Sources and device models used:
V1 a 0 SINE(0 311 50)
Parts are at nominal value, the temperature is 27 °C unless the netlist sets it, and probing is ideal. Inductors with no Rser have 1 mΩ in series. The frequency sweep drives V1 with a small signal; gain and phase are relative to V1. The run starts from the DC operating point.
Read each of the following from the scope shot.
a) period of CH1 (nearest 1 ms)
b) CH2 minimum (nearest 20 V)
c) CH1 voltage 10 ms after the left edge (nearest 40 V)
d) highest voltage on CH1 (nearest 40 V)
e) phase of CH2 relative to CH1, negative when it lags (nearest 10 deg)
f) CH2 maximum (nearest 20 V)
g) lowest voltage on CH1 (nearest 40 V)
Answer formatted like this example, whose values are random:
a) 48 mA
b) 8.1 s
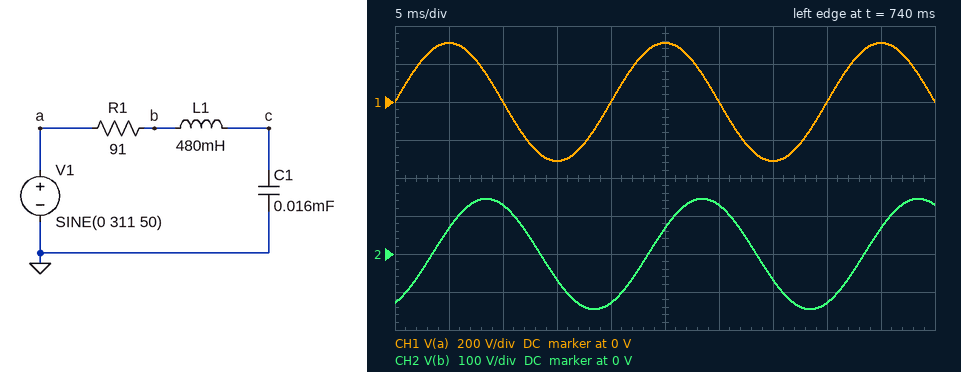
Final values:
a) 20 ms
b) -140 V
c) 0 V
d) 320 V
e) -60 deg
f) 140 V
g) -320 V
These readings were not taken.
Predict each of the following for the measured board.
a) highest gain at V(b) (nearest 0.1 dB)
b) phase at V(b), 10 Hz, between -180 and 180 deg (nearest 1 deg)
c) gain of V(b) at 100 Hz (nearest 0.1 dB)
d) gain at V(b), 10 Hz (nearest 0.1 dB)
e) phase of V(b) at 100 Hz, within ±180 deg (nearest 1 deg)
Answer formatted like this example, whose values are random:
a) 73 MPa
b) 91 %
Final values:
a) 0 dB
b) -5 deg
c) -0.8 dB
d) 0 dB
e) 24 deg
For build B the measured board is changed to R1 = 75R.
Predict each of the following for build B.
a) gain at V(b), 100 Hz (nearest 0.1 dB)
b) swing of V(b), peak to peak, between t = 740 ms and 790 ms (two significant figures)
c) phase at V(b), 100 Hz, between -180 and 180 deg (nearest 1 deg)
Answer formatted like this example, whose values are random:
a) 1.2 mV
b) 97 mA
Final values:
a) -0.6 dB
b) 340 V
c) 20 deg
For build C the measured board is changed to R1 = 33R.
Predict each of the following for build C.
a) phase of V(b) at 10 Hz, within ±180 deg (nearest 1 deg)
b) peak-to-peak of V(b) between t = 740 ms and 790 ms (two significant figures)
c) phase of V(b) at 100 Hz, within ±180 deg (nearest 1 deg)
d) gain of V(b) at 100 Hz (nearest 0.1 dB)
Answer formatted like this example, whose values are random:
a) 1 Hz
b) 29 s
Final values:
a) -2 deg
b) 510 V
c) 9 deg
d) -0.1 dB
